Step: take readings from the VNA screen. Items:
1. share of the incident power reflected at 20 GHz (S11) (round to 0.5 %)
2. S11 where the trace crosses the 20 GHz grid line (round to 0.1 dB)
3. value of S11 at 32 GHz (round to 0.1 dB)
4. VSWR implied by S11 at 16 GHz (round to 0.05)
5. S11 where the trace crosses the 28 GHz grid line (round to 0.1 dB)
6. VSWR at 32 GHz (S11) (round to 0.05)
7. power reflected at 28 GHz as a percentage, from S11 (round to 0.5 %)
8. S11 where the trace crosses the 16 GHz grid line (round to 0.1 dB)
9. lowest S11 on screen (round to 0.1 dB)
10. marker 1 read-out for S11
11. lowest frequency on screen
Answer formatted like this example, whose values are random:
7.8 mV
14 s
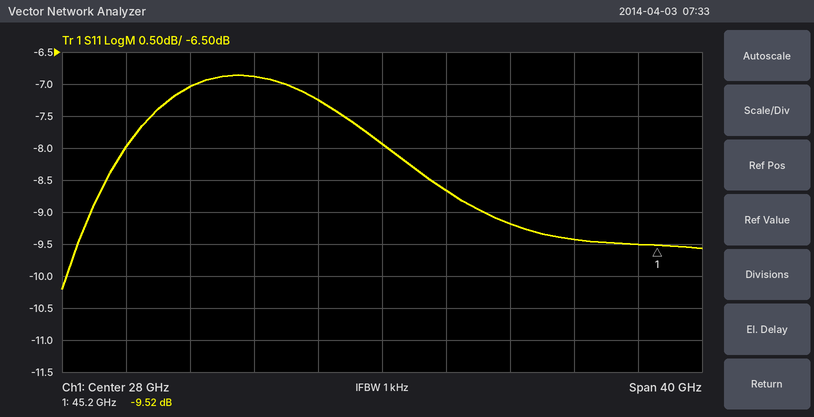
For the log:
20.5 %
-6.9 dB
-8.7 dB
2.60
-7.9 dB
2.15
16.0 %
-7.0 dB
-10.2 dB
-9.52 dB
8 GHz
